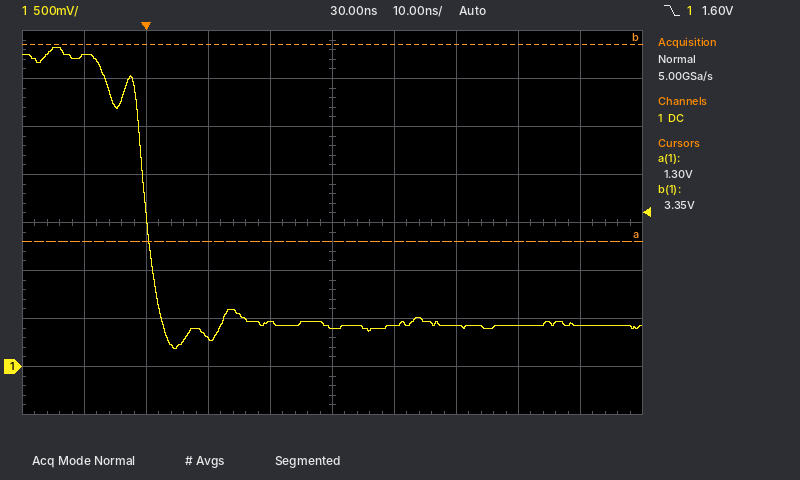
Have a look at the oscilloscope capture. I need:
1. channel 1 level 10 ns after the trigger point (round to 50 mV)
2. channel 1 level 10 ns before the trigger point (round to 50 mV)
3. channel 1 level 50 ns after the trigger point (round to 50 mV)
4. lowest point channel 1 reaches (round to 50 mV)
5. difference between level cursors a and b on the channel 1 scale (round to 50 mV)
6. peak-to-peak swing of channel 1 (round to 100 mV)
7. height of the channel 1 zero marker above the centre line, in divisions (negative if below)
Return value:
300 mV
3.25 V
450 mV
200 mV
2.05 V
3.10 V
-3.0 div
